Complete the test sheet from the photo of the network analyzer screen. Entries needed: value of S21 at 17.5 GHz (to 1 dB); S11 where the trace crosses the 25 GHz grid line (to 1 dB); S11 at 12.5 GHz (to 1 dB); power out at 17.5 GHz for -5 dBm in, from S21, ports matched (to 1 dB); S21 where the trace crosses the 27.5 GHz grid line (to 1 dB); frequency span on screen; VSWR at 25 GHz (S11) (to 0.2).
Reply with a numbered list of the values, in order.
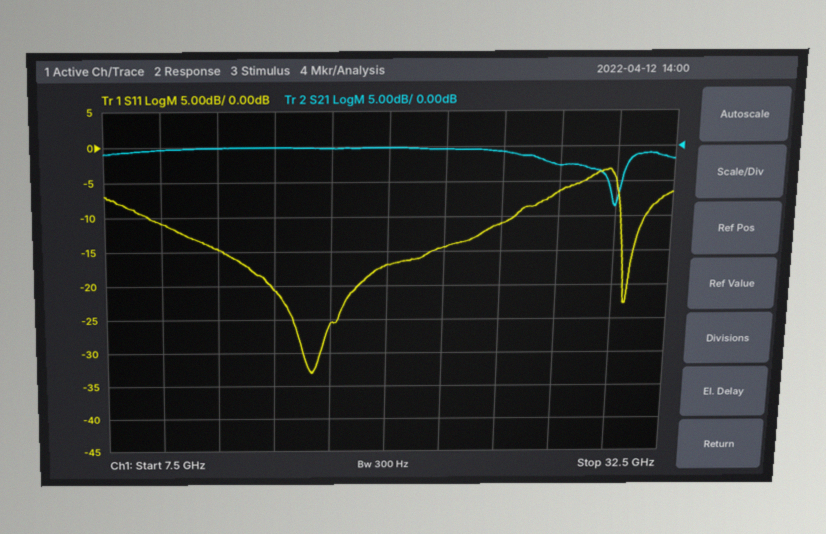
1. 0 dB
2. -11 dB
3. -15 dB
4. -5 dBm
5. -3 dB
6. 25 GHz
7. 1.8
